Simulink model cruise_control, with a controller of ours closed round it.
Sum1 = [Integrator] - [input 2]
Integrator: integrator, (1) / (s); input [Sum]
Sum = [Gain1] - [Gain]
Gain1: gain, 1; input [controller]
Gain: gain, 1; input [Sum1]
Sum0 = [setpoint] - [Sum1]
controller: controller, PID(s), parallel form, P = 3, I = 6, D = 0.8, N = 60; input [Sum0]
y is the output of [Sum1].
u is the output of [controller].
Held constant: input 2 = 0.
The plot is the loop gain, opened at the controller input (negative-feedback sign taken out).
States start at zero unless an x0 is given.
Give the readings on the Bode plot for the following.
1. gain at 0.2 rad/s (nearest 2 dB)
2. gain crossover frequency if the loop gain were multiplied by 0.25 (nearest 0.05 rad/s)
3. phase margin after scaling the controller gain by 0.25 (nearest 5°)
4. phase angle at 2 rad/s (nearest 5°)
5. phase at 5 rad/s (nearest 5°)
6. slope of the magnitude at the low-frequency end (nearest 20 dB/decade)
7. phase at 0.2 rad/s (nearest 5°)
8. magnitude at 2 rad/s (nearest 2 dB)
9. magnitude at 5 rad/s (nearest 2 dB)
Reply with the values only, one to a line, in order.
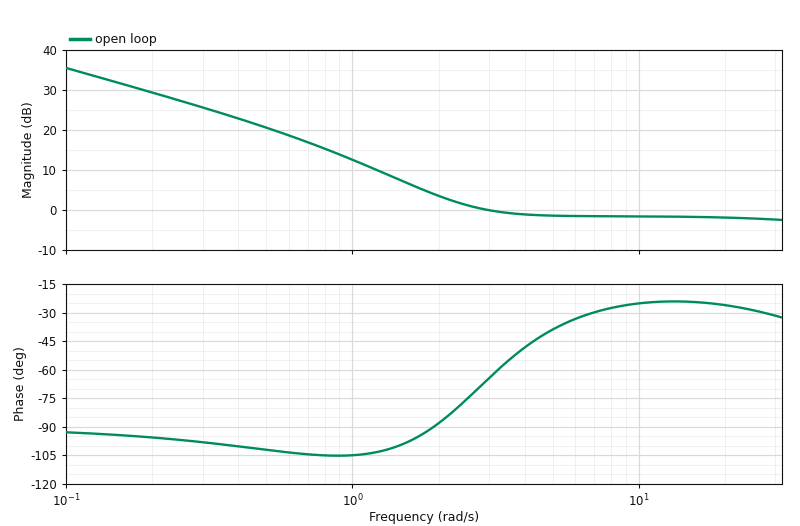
30 dB
1.05 rad/s
75°
-90°
-40°
-20 dB/decade
-95°
4 dB
-2 dB
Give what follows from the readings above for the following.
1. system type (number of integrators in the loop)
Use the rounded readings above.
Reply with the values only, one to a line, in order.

1
